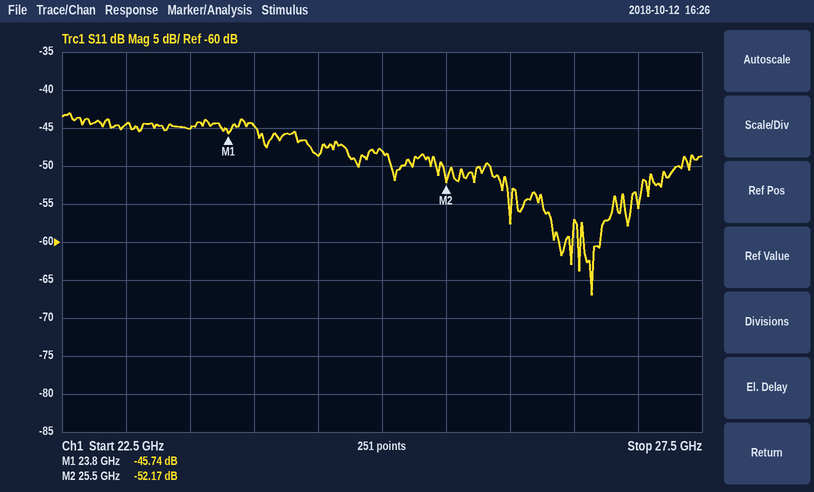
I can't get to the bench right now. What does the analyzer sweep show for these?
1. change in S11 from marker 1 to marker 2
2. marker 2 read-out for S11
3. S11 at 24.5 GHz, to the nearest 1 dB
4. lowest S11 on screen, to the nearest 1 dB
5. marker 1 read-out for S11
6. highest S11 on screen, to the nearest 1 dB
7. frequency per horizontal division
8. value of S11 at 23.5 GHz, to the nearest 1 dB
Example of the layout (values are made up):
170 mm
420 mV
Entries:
-6.43 dB
-52.17 dB
-49 dB
-67 dB
-45.74 dB
-43 dB
500 MHz
-45 dB
